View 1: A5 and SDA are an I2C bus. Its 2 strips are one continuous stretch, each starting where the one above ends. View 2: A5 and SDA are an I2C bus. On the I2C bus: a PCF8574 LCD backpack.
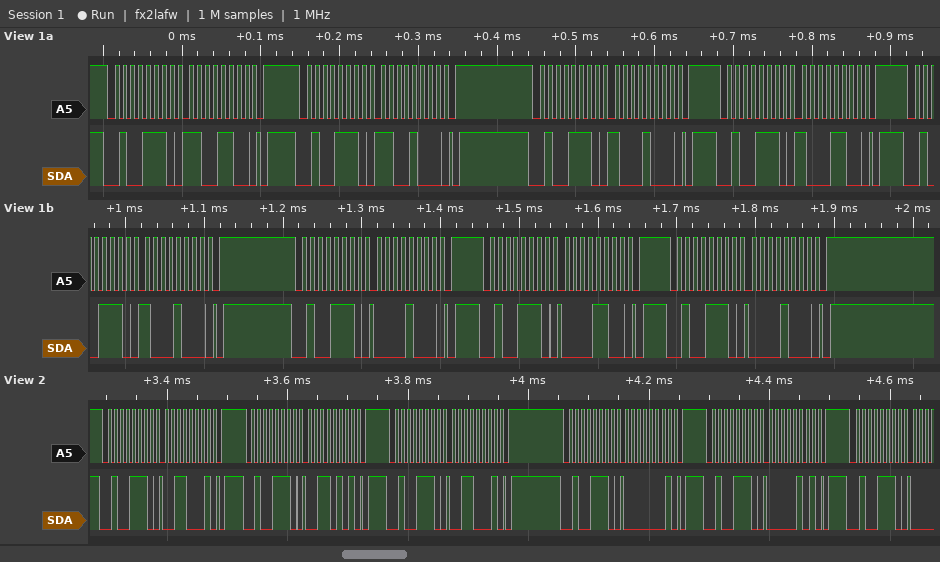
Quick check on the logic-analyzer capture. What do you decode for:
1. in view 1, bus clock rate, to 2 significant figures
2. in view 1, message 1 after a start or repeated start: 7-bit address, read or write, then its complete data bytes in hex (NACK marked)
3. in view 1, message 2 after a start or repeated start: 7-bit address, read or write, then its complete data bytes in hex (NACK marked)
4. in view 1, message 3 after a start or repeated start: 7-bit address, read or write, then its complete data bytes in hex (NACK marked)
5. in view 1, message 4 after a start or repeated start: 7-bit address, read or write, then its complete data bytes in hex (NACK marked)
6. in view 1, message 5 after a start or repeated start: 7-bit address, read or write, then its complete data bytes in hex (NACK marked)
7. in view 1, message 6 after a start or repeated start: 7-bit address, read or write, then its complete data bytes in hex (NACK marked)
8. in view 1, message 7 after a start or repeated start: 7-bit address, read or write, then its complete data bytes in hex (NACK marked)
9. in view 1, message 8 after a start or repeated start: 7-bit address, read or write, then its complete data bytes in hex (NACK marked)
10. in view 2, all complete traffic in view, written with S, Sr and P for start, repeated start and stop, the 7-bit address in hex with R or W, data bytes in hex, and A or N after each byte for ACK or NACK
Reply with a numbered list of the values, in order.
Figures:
1. 100 kHz
2. 0x27 write: CC
3. 0x27 write: C8
4. 0x27 write: 88
5. 0x27 write: 8C
6. 0x27 write: 88
7. 0x27 write: 08
8. 0x27 write: 0C
9. 0x27 write: 08
10. S 27W A 31 A P S 27W A 35 A P S 27W A 31 A P S 27W A 01 A P S 27W A 05 A P S 27W A
